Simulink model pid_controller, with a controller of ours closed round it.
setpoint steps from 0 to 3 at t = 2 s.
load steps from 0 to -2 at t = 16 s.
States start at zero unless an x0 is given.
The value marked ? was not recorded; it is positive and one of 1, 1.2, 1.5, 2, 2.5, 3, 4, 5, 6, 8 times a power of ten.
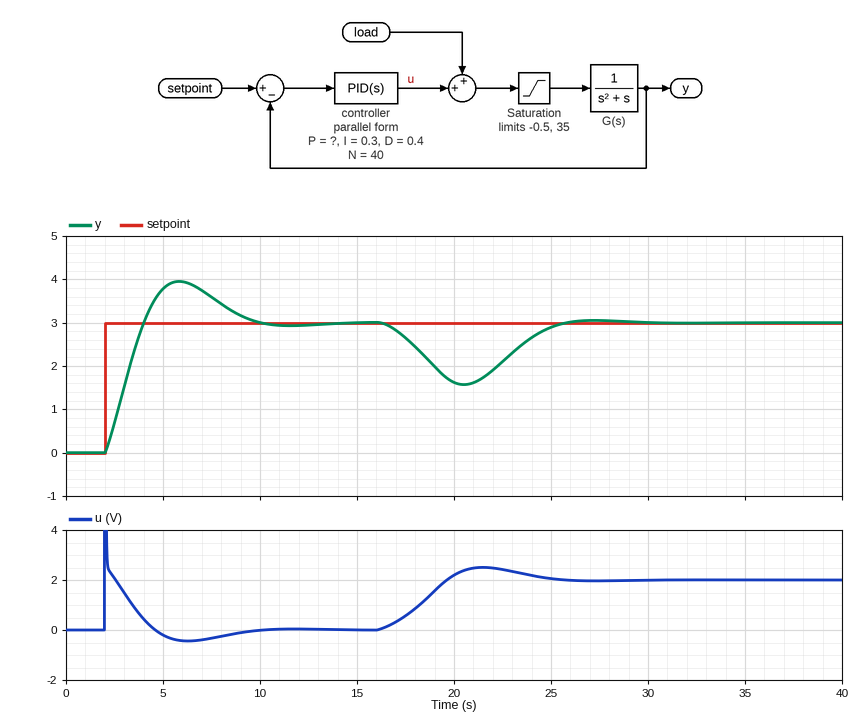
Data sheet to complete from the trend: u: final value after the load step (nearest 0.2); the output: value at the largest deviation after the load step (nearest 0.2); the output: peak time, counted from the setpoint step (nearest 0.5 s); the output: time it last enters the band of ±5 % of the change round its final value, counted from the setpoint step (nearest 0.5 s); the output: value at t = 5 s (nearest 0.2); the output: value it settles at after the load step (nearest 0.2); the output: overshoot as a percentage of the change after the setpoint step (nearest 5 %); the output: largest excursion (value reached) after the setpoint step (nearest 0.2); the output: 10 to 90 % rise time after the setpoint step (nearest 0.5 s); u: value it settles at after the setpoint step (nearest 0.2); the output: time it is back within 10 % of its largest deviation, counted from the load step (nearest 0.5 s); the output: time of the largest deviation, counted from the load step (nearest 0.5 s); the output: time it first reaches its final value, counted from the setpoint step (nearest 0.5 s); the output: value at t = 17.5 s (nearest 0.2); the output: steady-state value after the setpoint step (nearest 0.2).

2.0
1.6
4.0 s
7.0 s
3.8
3.0
30 %
4.0
1.5 s
0.0
9.0 s
4.5 s
2.0 s
2.6
3.0
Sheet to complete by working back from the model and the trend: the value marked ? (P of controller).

1
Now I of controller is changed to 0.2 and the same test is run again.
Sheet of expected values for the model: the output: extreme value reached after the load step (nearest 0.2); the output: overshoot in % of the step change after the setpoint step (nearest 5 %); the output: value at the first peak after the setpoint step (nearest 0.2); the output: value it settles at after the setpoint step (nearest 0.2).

1.4
25 %
3.8
3.0
